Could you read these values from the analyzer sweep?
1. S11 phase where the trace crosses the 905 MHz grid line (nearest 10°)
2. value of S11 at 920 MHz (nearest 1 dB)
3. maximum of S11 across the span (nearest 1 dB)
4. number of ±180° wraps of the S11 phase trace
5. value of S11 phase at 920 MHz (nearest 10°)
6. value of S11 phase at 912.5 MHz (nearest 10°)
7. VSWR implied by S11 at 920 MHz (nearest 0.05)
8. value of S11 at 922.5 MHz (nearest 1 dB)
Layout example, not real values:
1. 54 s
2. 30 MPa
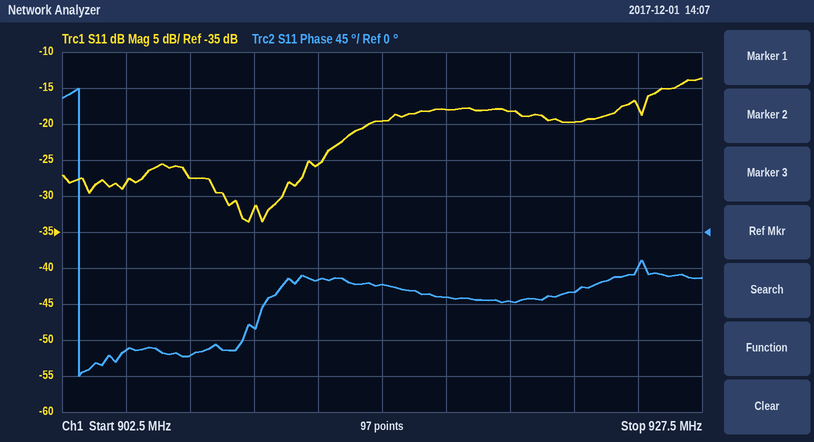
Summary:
1. -150°
2. -18 dB
3. -14 dB
4. 1
5. -90°
6. -60°
7. 1.30
8. -20 dB
